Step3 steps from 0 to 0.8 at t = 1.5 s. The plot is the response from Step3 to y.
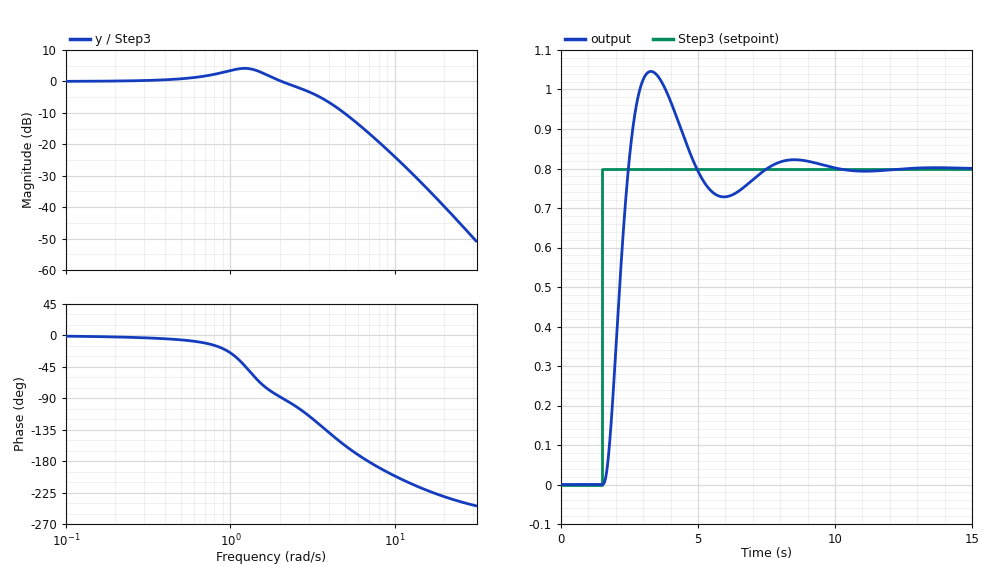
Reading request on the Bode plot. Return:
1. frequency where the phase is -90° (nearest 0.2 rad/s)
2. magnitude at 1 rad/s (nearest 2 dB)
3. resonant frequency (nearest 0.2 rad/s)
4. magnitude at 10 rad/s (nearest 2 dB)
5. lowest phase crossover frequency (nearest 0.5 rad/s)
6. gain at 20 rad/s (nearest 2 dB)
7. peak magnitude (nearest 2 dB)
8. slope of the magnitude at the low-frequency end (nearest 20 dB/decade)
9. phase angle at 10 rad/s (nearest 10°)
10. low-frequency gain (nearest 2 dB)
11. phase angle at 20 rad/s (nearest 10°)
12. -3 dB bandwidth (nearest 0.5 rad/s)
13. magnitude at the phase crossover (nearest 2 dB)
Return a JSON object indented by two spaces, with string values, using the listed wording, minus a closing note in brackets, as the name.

{
  "frequency where the phase is -90°": "2.0 rad/s",
  "magnitude at 1 rad/s": "4 dB",
  "resonant frequency": "1.2 rad/s",
  "magnitude at 10 rad/s": "-24 dB",
  "lowest phase crossover frequency": "7.0 rad/s",
  "gain at 20 rad/s": "-40 dB",
  "peak magnitude": "4 dB",
  "slope of the magnitude at the low-frequency end": "0 dB/decade",
  "phase angle at 10 rad/s": "-200°",
  "low-frequency gain": "0 dB",
  "phase angle at 20 rad/s": "-230°",
  "-3 dB bandwidth": "3.0 rad/s",
  "magnitude at the phase crossover": "-16 dB"
}
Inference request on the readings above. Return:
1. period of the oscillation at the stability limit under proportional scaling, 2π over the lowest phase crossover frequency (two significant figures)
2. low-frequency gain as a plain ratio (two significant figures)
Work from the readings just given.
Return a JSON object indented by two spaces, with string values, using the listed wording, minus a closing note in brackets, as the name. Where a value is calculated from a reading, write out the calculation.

{
  "period of the oscillation at the stability limit under proportional scaling, 2π over the lowest phase crossover frequency": "2π / 7 = 0.90 s",
  "low-frequency gain as a plain ratio": "10^(0 / 20) = 1.0"
}
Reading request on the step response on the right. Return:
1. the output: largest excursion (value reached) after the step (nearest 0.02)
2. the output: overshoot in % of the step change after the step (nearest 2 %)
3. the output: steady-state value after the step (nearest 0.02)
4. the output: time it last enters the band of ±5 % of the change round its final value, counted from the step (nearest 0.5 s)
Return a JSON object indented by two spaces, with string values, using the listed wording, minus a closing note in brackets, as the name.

{
  "the output: largest excursion (value reached) after the step": "1.04",
  "the output: overshoot in % of the step change after the step": "30 %",
  "the output: steady-state value after the step": "0.80",
  "the output: time it last enters the band of ±5 % of the change round its final value, counted from the step": "5.5 s"
}
